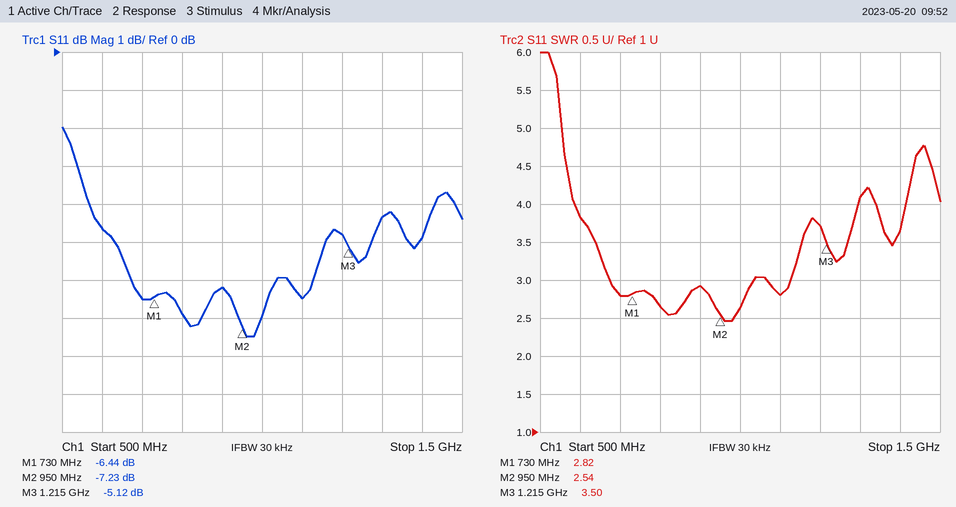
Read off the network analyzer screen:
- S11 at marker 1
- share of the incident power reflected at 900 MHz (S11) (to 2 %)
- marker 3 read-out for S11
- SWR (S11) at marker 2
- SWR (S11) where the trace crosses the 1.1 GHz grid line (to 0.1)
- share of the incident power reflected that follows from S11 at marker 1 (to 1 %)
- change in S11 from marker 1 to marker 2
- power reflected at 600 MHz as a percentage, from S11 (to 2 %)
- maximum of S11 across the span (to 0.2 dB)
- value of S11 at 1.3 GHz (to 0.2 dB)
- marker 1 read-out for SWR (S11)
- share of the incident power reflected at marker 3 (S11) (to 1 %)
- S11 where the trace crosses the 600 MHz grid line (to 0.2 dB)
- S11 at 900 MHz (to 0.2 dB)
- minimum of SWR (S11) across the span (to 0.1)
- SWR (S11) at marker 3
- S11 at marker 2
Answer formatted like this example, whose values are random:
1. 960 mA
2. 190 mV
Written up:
1. -6.44 dB
2. 24 %
3. -5.12 dB
4. 2.54
5. 2.8
6. 23 %
7. -0.79 dB
8. 34 %
9. -2.0 dB
10. -4.4 dB
11. 2.82
12. 31 %
13. -4.6 dB
14. -6.2 dB
15. 2.5
16. 3.50
17. -7.23 dB
